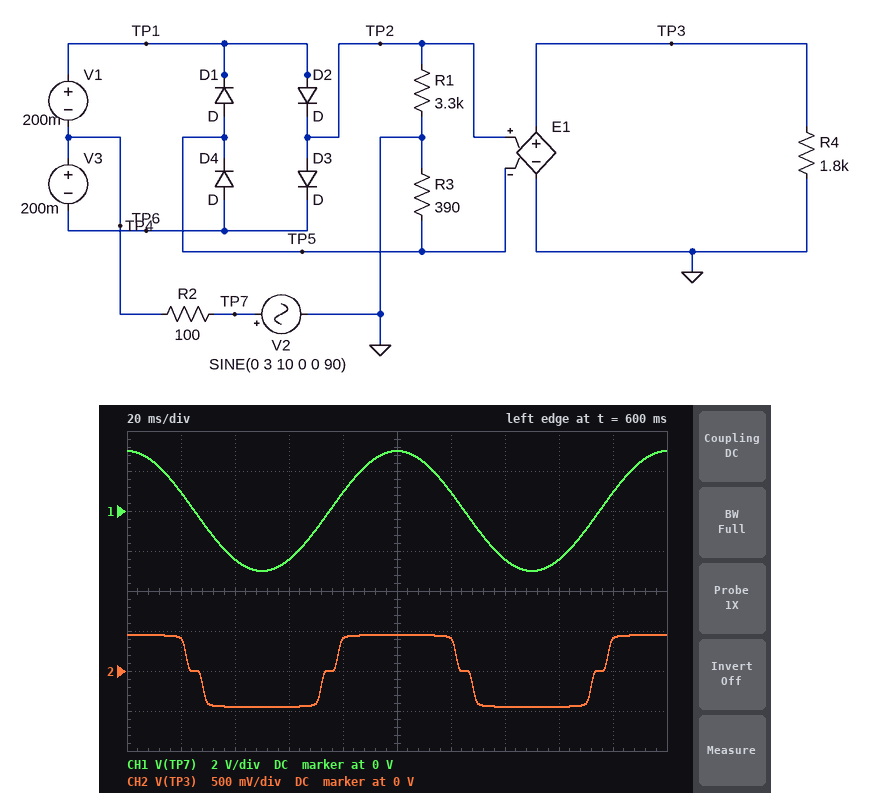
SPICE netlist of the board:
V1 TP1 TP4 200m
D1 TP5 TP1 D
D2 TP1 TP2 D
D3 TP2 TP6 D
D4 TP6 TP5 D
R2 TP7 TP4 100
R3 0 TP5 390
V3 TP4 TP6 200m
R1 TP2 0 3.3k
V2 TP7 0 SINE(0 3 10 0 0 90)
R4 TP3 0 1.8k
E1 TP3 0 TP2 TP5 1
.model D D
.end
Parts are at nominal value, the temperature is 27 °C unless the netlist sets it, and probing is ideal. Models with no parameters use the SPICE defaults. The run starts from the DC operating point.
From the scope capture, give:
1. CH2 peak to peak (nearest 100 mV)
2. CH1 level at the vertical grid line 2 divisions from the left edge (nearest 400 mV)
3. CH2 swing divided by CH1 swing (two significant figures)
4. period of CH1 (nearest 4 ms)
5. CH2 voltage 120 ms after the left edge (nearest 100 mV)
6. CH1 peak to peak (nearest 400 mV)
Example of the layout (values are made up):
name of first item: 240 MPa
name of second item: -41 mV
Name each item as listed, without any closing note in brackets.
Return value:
CH2 peak to peak: 900 mV
CH1 level at the vertical grid line 2 divisions from the left edge: -2.4 V
CH2 swing divided by CH1 swing: 0.15
period of CH1: 100 ms
CH2 voltage 120 ms after the left edge: 400 mV
CH1 peak to peak: 6.0 V
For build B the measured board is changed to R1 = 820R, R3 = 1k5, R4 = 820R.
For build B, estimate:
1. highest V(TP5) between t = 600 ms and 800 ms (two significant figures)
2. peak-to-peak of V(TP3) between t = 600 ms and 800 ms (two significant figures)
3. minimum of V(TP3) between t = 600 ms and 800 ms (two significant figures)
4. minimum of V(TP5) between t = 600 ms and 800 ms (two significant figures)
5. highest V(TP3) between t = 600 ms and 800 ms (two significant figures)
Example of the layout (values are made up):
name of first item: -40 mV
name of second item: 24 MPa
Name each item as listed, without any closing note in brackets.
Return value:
highest V(TP5) between t = 600 ms and 800 ms: 1.8 V
peak-to-peak of V(TP3) between t = 600 ms and 800 ms: 760 mV
minimum of V(TP3) between t = 600 ms and 800 ms: -380 mV
minimum of V(TP5) between t = 600 ms and 800 ms: -1.8 V
highest V(TP3) between t = 600 ms and 800 ms: 380 mV
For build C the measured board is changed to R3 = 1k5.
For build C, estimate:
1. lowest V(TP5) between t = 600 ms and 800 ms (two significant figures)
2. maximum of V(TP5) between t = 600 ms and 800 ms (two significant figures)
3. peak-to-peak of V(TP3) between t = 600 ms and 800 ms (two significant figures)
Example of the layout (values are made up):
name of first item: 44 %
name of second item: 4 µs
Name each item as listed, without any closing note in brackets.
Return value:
lowest V(TP5) between t = 600 ms and 800 ms: -1.9 V
maximum of V(TP5) between t = 600 ms and 800 ms: 1.9 V
peak-to-peak of V(TP3) between t = 600 ms and 800 ms: 830 mV
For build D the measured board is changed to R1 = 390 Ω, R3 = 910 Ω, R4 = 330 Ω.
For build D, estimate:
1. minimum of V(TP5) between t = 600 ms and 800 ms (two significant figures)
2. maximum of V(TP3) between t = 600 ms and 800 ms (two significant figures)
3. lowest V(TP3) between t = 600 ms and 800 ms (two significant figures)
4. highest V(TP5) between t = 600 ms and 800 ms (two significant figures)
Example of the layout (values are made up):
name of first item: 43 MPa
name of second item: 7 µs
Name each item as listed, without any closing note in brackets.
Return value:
minimum of V(TP5) between t = 600 ms and 800 ms: -1.5 V
maximum of V(TP3) between t = 600 ms and 800 ms: 370 mV
lowest V(TP3) between t = 600 ms and 800 ms: -370 mV
highest V(TP5) between t = 600 ms and 800 ms: 1.5 V
